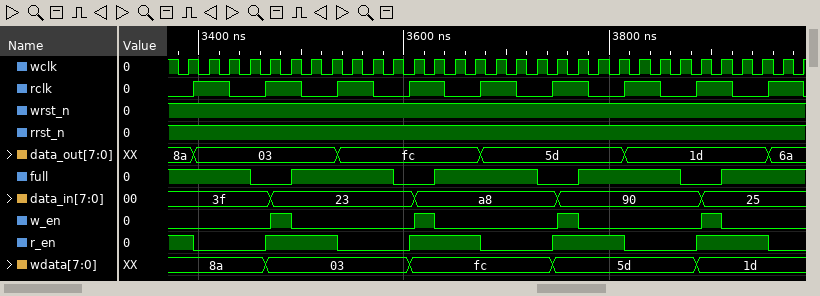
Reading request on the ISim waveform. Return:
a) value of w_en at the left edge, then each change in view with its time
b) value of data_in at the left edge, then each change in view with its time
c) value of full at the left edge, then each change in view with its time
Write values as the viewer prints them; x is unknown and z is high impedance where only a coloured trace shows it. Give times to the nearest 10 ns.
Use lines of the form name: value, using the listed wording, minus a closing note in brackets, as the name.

value of w_en at the left edge, then each change in view with its time: 0, 1 at 3470 ns, 0 at 3490 ns, 1 at 3610 ns, 0 at 3630 ns, 1 at 3750 ns, 0 at 3770 ns, 1 at 3890 ns, 0 at 3910 ns
value of data_in at the left edge, then each change in view with its time: 3f, 23 at 3470 ns, a8 at 3610 ns, 90 at 3750 ns, 25 at 3890 ns
value of full at the left edge, then each change in view with its time: 1, 0 at 3450 ns, 1 at 3490 ns, 0 at 3590 ns, 1 at 3630 ns, 0 at 3730 ns, 1 at 3770 ns, 0 at 3870 ns, 1 at 3910 ns
